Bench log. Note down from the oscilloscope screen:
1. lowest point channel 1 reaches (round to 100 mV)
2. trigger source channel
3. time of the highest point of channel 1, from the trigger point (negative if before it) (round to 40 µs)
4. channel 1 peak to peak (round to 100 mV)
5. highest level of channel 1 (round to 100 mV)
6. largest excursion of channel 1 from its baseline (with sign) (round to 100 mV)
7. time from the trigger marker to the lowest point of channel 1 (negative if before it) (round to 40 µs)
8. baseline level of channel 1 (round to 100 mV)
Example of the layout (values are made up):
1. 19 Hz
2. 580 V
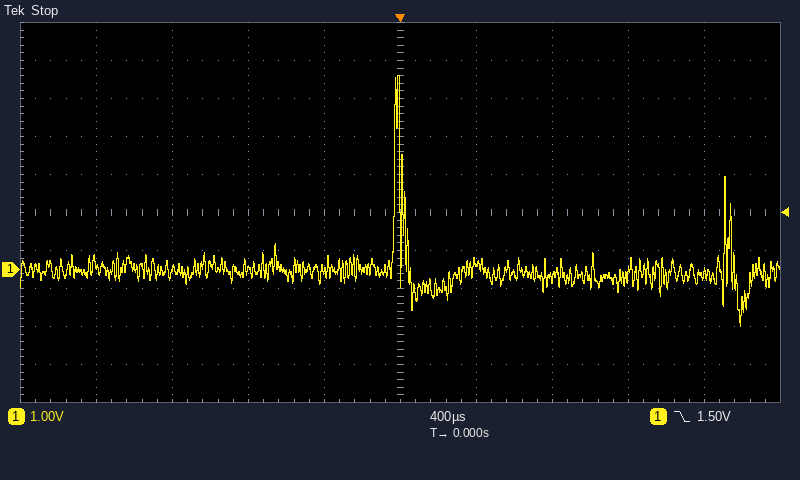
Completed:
1. -1.5 V
2. channel 1
3. 0 µs
4. 6.6 V
5. 5.1 V
6. +5.2 V
7. +1.80 ms
8. -100 mV
